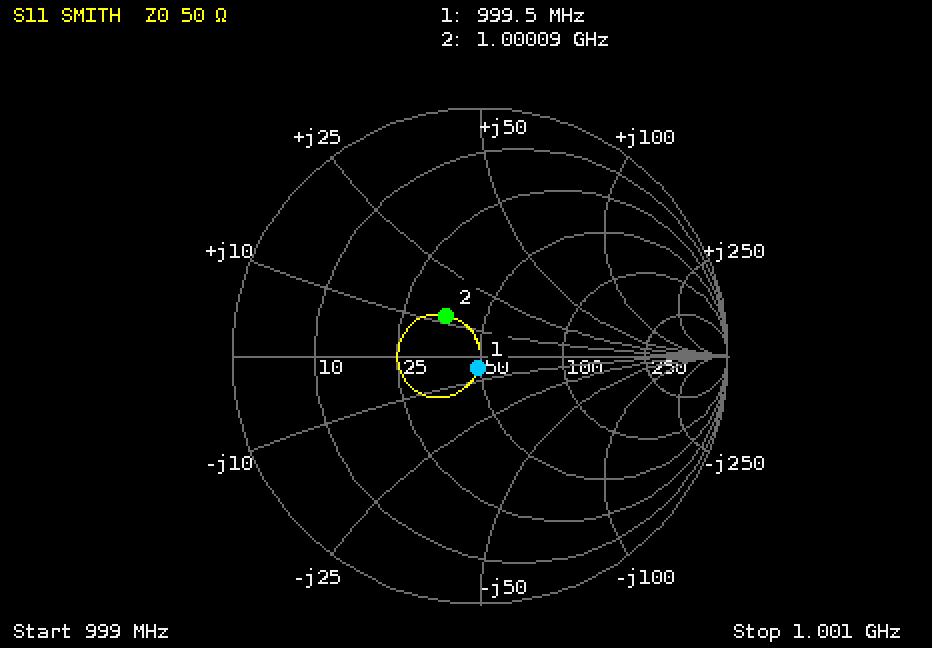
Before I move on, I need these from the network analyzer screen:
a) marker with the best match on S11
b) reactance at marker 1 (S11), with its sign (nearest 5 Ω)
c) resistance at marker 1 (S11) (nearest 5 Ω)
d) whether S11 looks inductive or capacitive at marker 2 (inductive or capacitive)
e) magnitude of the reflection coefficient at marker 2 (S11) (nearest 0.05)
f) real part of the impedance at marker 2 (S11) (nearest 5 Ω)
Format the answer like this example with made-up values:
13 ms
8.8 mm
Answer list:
marker 1
-5 Ω
50 Ω
inductive
0.20
35 Ω
